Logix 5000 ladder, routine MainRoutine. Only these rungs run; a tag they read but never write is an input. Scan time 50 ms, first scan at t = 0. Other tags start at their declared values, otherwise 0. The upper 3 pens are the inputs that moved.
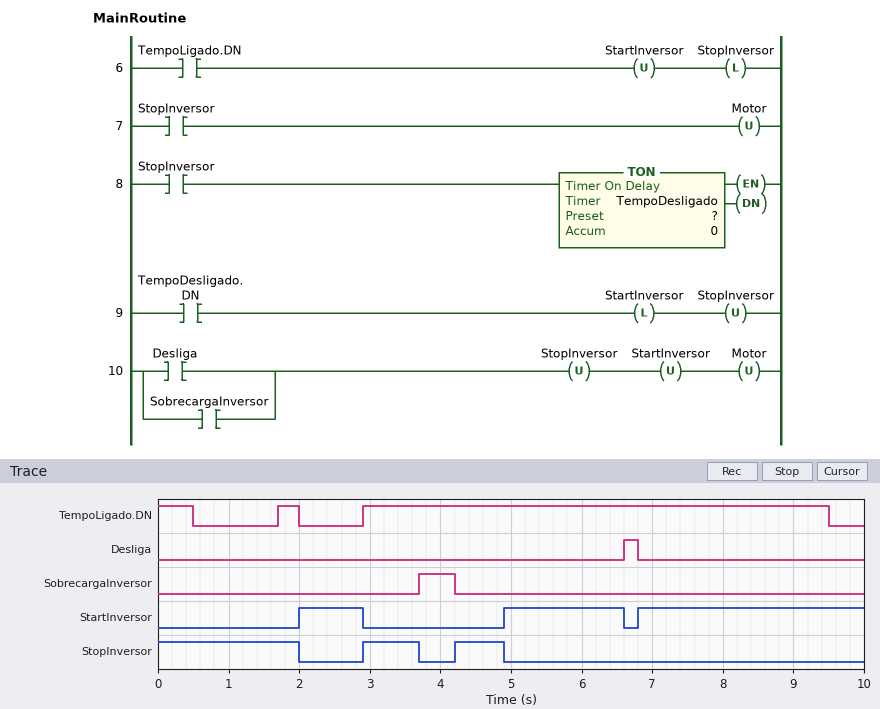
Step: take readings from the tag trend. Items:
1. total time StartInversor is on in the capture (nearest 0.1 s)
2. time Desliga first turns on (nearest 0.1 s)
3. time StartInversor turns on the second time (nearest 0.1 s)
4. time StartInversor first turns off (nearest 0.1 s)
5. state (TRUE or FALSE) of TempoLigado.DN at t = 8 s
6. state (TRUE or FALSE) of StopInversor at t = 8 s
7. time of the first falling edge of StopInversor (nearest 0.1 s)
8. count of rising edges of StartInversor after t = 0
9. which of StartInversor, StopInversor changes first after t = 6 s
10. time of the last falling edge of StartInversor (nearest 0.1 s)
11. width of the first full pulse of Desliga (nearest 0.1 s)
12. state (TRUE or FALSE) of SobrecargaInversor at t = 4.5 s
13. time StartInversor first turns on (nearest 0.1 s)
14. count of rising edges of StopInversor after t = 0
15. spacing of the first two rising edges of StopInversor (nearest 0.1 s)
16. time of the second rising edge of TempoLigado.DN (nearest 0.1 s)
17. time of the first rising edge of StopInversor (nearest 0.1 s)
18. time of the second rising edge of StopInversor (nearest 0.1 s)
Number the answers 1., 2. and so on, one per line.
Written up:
1. 5.8 s
2. 6.6 s
3. 4.9 s
4. 2.9 s
5. TRUE
6. FALSE
7. 2.0 s
8. 3
9. StartInversor
10. 6.6 s
11. 0.2 s
12. FALSE
13. 2.0 s
14. 2
15. 1.3 s
16. 2.9 s
17. 2.9 s
18. 4.2 s
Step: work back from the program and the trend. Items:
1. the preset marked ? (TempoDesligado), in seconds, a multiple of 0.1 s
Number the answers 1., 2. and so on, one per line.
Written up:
1. 2.0 s
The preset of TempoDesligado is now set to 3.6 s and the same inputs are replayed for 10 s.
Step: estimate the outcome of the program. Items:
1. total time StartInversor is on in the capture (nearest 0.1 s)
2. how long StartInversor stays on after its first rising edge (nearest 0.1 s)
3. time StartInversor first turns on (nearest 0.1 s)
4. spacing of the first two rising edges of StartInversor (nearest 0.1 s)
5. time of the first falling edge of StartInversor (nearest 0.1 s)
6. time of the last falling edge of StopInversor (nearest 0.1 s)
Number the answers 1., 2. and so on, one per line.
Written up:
1. 5.7 s
2. 0.1 s
3. 3.6 s
4. 0.6 s
5. 3.7 s
6. 3.6 s
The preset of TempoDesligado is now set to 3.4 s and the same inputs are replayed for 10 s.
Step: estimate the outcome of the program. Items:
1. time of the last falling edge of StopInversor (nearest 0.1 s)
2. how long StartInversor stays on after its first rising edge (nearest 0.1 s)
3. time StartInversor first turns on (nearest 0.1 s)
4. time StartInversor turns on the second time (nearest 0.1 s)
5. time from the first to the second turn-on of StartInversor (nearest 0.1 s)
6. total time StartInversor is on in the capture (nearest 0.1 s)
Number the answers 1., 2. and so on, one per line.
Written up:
1. 3.4 s
2. 0.3 s
3. 3.4 s
4. 4.2 s
5. 0.8 s
6. 5.9 s
